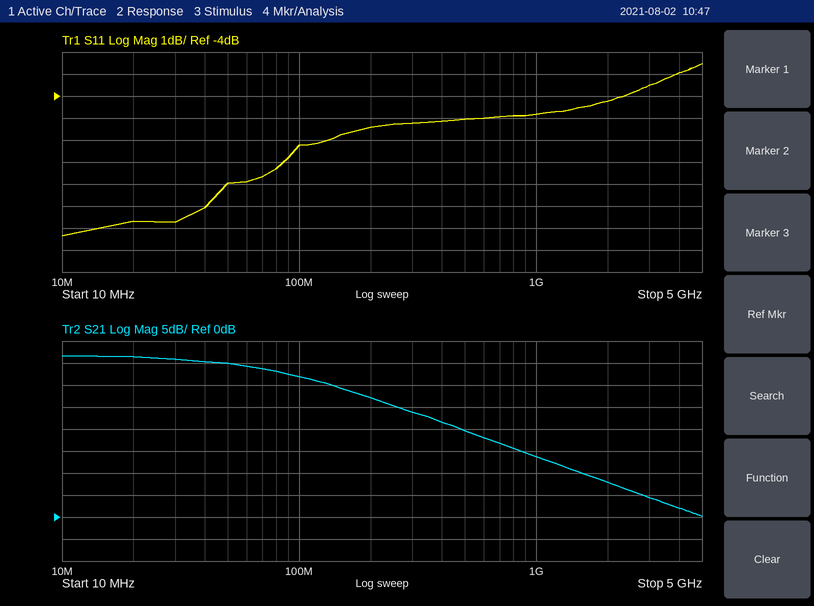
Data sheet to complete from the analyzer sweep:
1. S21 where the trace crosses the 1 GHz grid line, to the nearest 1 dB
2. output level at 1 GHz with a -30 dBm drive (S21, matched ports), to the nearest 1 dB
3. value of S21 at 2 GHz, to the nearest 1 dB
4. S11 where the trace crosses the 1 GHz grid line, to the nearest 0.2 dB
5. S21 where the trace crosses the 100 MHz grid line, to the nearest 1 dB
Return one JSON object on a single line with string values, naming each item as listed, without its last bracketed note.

{"S21 where the trace crosses the 1 GHz grid line, to the nearest 1 dB": "14 dB", "output level at 1 GHz with a -30 dBm drive (S21, matched ports), to the nearest 1 dB": "-16 dBm", "value of S21 at 2 GHz, to the nearest 1 dB": "8 dB", "S11 where the trace crosses the 1 GHz grid line, to the nearest 0.2 dB": "-4.8 dB", "S21 where the trace crosses the 100 MHz grid line, to the nearest 1 dB": "32 dB"}
